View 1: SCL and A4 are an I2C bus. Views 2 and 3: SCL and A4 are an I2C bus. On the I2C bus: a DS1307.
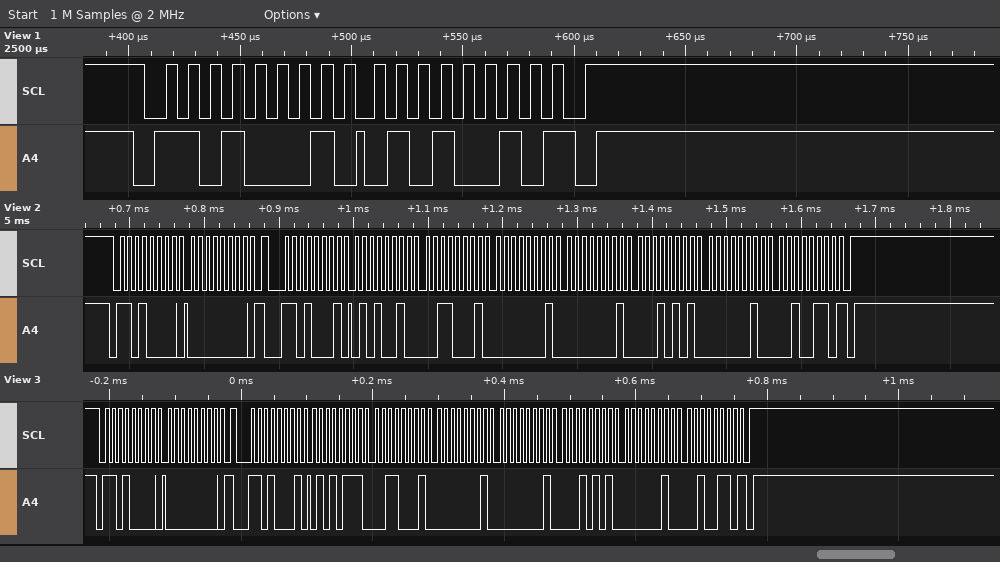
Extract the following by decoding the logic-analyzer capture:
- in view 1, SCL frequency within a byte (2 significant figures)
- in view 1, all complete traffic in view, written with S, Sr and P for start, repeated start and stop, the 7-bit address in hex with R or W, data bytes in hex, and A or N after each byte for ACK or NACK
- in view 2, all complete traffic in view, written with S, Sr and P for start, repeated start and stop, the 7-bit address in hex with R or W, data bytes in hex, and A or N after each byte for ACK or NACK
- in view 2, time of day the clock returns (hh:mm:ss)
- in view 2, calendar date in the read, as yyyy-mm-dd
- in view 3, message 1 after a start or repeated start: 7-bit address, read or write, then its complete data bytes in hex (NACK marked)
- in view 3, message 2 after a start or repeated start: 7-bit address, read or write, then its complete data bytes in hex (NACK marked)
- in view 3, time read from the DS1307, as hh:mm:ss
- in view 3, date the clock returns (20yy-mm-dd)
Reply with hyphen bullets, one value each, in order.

- 100 kHz
- S 68R A 52 N P
- S 68W A 00 A Sr 68R A 52 A 31 A 01 A 01 A 15 A 02 A 26 N P
- 01:31:52
- 2026-02-15
- 0x68 write: 00
- 0x68 read: 57 31 01 01 15 02 26 NACK
- 01:31:57
- 2026-02-15
